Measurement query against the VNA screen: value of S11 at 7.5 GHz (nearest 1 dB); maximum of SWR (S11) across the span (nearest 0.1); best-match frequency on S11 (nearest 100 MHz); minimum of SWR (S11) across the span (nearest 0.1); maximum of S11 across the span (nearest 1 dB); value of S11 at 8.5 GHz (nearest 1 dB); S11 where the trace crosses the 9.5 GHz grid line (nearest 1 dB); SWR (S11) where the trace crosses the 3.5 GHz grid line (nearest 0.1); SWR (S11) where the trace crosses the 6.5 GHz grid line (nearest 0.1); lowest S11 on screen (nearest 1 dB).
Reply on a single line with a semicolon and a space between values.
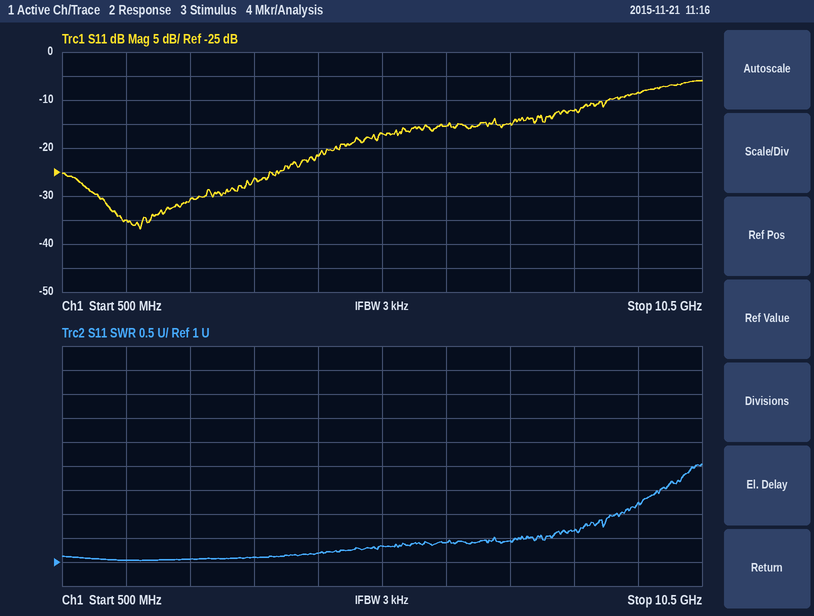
-15 dB; 3.0; 1.7 GHz; 1.0; -6 dB; -12 dB; -8 dB; 1.1; 1.4; -37 dB
